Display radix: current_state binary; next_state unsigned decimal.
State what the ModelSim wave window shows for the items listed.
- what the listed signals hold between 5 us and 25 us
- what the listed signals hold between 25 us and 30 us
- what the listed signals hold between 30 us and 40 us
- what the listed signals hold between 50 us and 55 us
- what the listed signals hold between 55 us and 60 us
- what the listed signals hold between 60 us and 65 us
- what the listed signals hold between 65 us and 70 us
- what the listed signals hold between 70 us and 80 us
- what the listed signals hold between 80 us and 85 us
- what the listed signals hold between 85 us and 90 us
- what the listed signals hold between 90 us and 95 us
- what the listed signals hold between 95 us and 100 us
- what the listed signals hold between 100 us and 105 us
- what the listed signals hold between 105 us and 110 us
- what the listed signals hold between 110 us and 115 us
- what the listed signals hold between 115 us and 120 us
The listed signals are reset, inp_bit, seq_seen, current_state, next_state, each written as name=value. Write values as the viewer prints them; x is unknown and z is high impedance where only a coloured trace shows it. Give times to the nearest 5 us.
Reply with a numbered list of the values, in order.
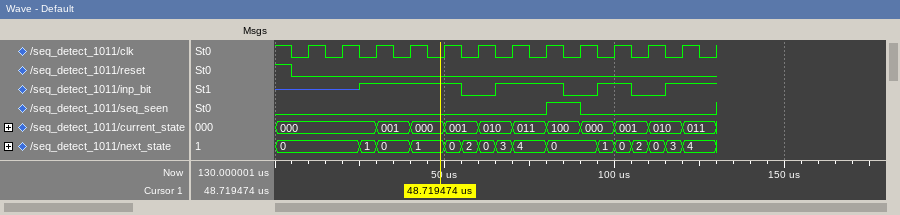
1. reset=0, inp_bit=z, seq_seen=0, current_state=000, next_state=0
2. reset=0, inp_bit=1, seq_seen=0, current_state=000, next_state=1
3. reset=0, inp_bit=1, seq_seen=0, current_state=001, next_state=0
4. reset=0, inp_bit=1, seq_seen=0, current_state=001, next_state=0
5. reset=0, inp_bit=0, seq_seen=0, current_state=001, next_state=2
6. reset=0, inp_bit=0, seq_seen=0, current_state=010, next_state=0
7. reset=0, inp_bit=1, seq_seen=0, current_state=010, next_state=3
8. reset=0, inp_bit=1, seq_seen=0, current_state=011, next_state=4
9. reset=0, inp_bit=1, seq_seen=1, current_state=100, next_state=0
10. reset=0, inp_bit=0, seq_seen=1, current_state=100, next_state=0
11. reset=0, inp_bit=0, seq_seen=0, current_state=000, next_state=0
12. reset=0, inp_bit=1, seq_seen=0, current_state=000, next_state=1
13. reset=0, inp_bit=1, seq_seen=0, current_state=001, next_state=0
14. reset=0, inp_bit=0, seq_seen=0, current_state=001, next_state=2
15. reset=0, inp_bit=0, seq_seen=0, current_state=010, next_state=0
16. reset=0, inp_bit=1, seq_seen=0, current_state=010, next_state=3
